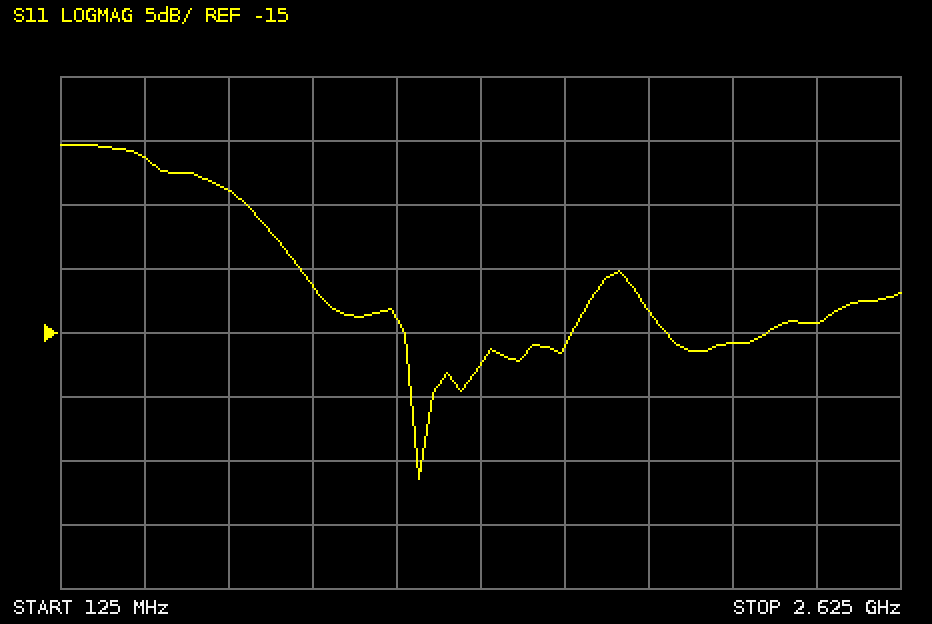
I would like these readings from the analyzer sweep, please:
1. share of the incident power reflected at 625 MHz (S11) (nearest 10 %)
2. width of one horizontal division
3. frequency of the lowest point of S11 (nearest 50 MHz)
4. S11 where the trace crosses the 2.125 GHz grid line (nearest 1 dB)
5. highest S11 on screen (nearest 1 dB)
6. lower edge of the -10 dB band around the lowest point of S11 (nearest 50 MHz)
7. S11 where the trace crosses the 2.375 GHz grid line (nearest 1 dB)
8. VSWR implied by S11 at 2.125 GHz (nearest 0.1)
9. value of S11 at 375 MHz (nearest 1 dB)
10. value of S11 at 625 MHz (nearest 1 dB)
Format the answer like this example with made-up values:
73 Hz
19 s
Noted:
40 %
250 MHz
1.20 GHz
-16 dB
0 dB
850 MHz
-14 dB
1.4
-1 dB
-4 dB
